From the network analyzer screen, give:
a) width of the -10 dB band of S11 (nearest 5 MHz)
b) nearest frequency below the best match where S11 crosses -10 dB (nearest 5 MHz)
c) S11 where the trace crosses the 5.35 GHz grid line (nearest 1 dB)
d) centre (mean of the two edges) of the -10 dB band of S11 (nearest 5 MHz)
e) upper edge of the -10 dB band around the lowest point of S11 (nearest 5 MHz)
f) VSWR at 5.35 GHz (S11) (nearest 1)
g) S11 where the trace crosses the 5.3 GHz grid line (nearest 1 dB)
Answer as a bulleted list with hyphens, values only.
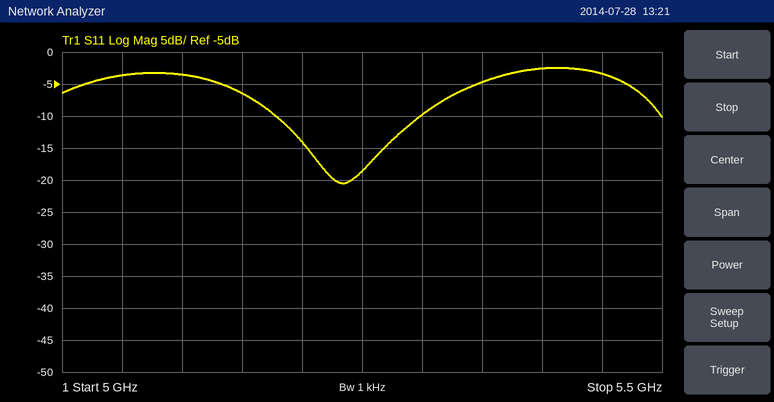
- 120 MHz
- 5.180 GHz
- -5 dB
- 5.240 GHz
- 5.300 GHz
- 4
- -10 dB
